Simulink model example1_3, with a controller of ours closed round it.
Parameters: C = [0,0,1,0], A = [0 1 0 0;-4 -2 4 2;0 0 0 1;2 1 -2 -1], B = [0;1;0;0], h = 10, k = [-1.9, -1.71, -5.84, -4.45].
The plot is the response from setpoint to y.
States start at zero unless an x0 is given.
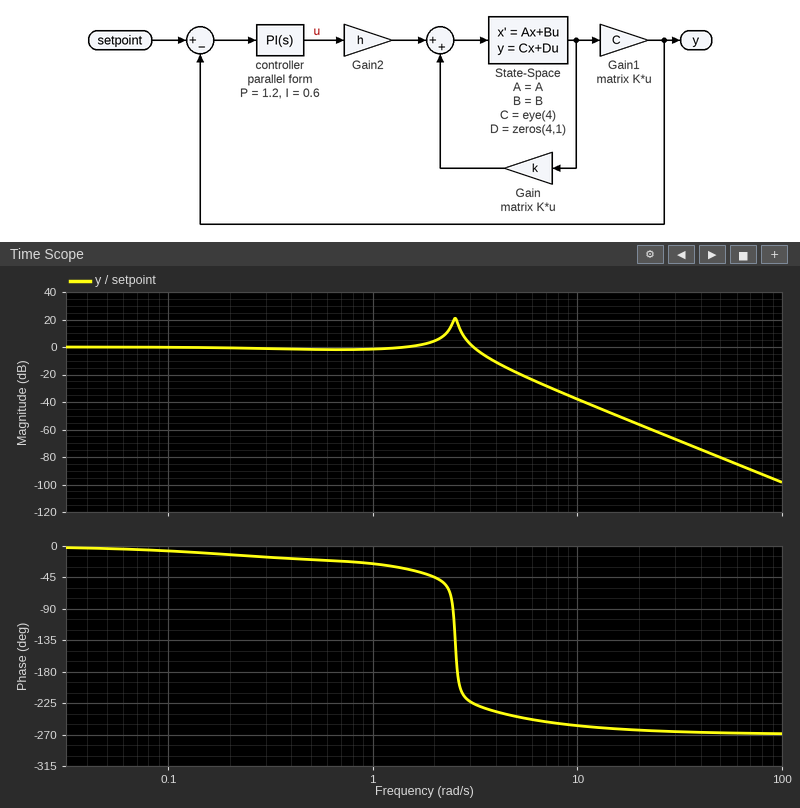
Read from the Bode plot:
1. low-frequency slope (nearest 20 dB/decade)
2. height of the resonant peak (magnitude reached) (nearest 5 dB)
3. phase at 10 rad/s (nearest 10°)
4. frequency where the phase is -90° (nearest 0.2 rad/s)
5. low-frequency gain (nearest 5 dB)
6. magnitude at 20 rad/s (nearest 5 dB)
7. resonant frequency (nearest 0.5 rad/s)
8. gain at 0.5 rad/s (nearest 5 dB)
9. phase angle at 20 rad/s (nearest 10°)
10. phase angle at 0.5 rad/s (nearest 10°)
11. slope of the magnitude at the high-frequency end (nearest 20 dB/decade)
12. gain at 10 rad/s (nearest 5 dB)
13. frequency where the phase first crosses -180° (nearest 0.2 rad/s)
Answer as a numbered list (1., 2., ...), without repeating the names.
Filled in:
1. 0 dB/decade
2. 20 dB
3. -260°
4. 2.4 rad/s
5. 0 dB
6. -55 dB
7. 2.5 rad/s
8. 0 dB
9. -260°
10. -20°
11. -60 dB/decade
12. -40 dB
13. 2.6 rad/s
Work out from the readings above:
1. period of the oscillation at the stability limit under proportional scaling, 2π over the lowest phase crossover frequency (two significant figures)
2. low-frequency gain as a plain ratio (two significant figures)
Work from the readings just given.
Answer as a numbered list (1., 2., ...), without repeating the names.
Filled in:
1. 2.4 s
2. 1.0
